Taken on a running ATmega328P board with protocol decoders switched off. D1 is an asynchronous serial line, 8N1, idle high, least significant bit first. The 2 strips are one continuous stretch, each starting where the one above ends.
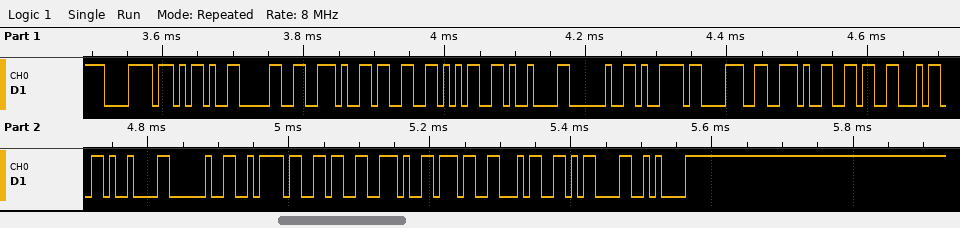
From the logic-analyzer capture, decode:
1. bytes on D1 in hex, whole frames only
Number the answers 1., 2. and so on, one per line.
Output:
1. 0x78 0x2D 0x30 0x2E 0x33 0x35 0x09 0x20 0x79 0x38 0x2E 0x36 0x34 0x09 0x20 0x7A 0x36 0x2E 0x37 0x34 0x0D 0x0A
